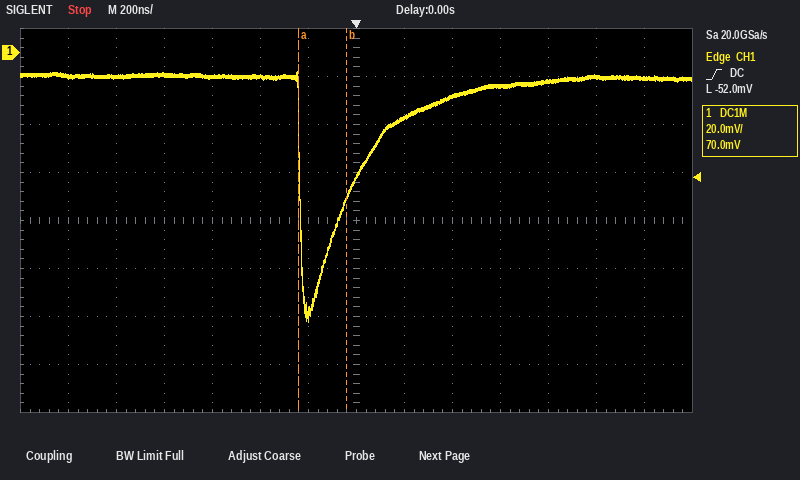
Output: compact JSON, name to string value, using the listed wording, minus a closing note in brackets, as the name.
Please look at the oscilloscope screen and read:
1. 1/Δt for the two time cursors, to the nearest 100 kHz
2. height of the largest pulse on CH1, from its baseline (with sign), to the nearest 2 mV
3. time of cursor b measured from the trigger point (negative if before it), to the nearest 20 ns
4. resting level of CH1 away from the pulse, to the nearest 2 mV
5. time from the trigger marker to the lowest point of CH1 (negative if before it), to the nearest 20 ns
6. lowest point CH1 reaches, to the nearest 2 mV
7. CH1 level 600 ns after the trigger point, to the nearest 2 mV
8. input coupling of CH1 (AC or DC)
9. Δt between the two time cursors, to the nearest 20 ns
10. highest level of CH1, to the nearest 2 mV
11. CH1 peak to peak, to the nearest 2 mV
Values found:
{"1/Δt for the two time cursors, to the nearest 100 kHz": "5.0 MHz", "height of the largest pulse on CH1, from its baseline (with sign), to the nearest 2 mV": "-102 mV", "time of cursor b measured from the trigger point (negative if before it), to the nearest 20 ns": "-40 ns", "resting level of CH1 away from the pulse, to the nearest 2 mV": "-10 mV", "time from the trigger marker to the lowest point of CH1 (negative if before it), to the nearest 20 ns": "-200 ns", "lowest point CH1 reaches, to the nearest 2 mV": "-112 mV", "CH1 level 600 ns after the trigger point, to the nearest 2 mV": "-14 mV", "input coupling of CH1": "DC", "Δt between the two time cursors, to the nearest 20 ns": "200 ns", "highest level of CH1, to the nearest 2 mV": "-8 mV", "CH1 peak to peak, to the nearest 2 mV": "104 mV"}
